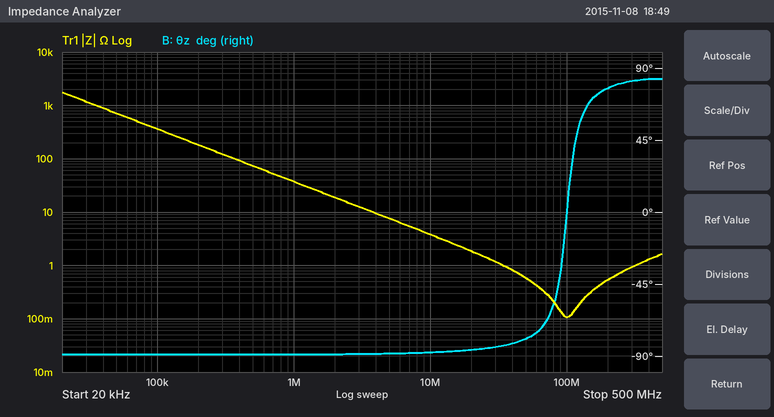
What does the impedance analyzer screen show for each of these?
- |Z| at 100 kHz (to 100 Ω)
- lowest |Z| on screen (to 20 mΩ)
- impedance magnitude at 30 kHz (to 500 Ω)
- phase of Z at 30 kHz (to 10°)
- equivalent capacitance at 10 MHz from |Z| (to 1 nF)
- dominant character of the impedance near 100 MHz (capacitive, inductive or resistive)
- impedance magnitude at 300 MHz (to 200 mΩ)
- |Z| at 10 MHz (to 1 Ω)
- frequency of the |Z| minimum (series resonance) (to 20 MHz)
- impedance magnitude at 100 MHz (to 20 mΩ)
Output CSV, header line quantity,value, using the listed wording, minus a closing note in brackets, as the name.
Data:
quantity,value
|Z| at 100 kHz,400 Ω
lowest |Z| on screen,100 mΩ
impedance magnitude at 30 kHz,1.0 kΩ
phase of Z at 30 kHz,-90°
equivalent capacitance at 10 MHz from |Z|,4 nF
dominant character of the impedance near 100 MHz,resistive
impedance magnitude at 300 MHz,1.0 Ω
|Z| at 10 MHz,4 Ω
frequency of the |Z| minimum (series resonance),100 MHz
impedance magnitude at 100 MHz,100 mΩ
